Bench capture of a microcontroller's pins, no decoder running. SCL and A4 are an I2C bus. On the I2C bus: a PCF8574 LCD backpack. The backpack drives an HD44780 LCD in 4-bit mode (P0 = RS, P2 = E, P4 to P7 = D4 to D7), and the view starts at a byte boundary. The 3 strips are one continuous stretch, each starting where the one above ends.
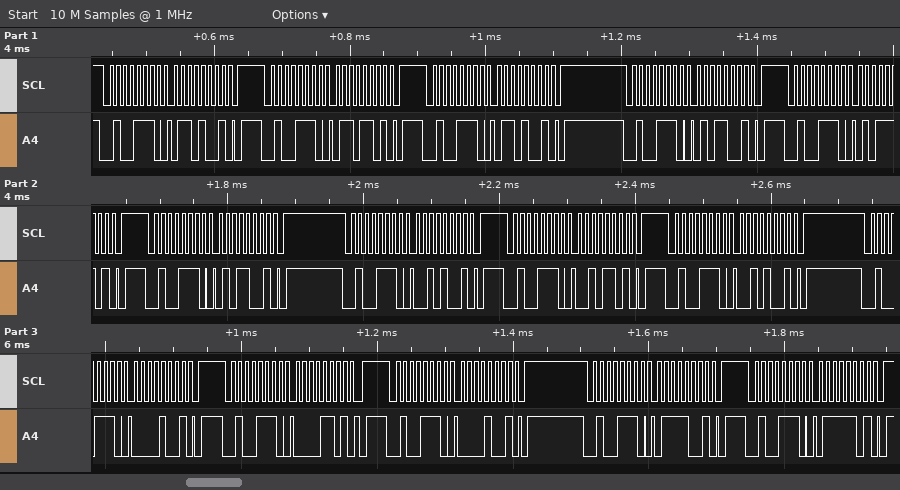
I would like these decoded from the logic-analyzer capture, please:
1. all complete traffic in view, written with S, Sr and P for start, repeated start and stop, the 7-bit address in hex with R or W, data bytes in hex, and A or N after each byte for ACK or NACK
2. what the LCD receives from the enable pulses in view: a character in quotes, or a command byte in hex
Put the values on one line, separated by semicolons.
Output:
S 27W A 69 A P S 27W A 6D A P S 27W A 69 A P S 27W A 59 A P S 27W A 5D A P S 27W A 59 A P S 27W A 29 A P S 27W A 2D A P S 27W A 29 A P S 27W A 09 A P S 27W A 0D A P S 27W A 09 A P S 27W A 79 A P S 27W A 7D A P; 'e' ' '
